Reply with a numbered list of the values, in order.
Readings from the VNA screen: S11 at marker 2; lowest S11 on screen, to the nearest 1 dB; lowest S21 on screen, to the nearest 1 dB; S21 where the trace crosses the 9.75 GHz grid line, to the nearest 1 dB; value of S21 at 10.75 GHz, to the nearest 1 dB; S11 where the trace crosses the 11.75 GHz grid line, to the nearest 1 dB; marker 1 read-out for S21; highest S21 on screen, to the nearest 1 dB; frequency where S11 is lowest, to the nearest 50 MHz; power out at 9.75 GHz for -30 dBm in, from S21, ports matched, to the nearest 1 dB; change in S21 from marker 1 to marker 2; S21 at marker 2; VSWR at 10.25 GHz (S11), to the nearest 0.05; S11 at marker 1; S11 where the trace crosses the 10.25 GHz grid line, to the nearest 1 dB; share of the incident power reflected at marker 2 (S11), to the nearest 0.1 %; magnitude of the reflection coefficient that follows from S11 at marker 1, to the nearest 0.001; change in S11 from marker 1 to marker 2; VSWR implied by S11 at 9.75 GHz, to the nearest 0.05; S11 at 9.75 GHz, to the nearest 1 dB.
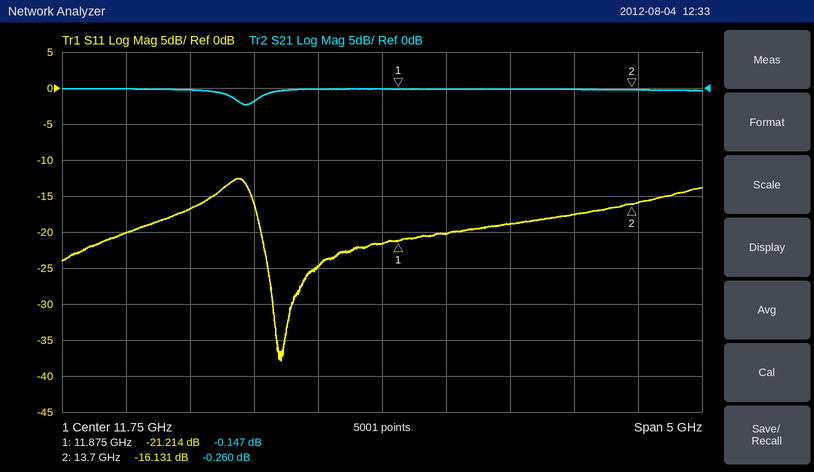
1. -16.131 dB
2. -38 dB
3. -2 dB
4. 0 dB
5. -2 dB
6. -22 dB
7. -0.147 dB
8. 0 dB
9. 10.95 GHz
10. -30 dBm
11. -0.113 dB
12. -0.260 dB
13. 1.35
14. -21.214 dB
15. -17 dB
16. 2.4 %
17. 0.087
18. 5.083 dB
19. 1.20
20. -20 dB
